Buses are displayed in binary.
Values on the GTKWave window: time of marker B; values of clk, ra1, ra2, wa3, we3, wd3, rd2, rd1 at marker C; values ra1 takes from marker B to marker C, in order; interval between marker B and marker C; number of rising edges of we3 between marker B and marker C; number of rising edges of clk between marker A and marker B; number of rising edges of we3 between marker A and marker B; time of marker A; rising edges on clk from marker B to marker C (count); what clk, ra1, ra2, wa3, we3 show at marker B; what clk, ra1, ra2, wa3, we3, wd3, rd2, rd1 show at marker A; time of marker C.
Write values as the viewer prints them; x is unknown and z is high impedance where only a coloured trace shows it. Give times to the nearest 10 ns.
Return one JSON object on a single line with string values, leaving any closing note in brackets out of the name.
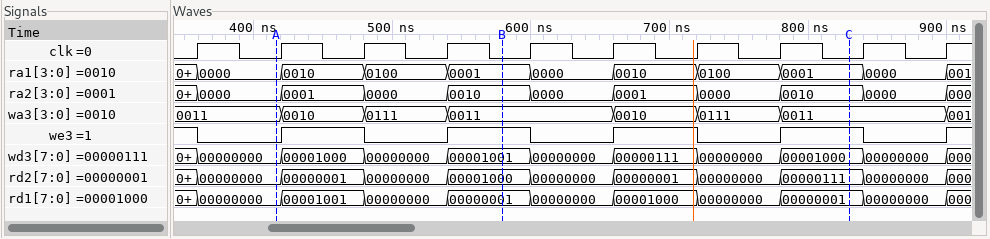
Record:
{"time of marker B": "580 ns", "values of clk, ra1, ra2, wa3, we3, wd3, rd2, rd1 at marker C": "clk=0, ra1=0001, ra2=0010, wa3=0011, we3=1, wd3=00001000, rd2=00000111, rd1=00000001", "values ra1 takes from marker B to marker C, in order": "0001, 0000, 0010, 0100, 0001", "interval between marker B and marker C": "250 ns", "number of rising edges of we3 between marker B and marker C": "2", "number of rising edges of clk between marker A and marker B": "3", "number of rising edges of we3 between marker A and marker B": "2", "time of marker A": "420 ns", "rising edges on clk from marker B to marker C": "4", "what clk, ra1, ra2, wa3, we3 show at marker B": "clk=0, ra1=0001, ra2=0010, wa3=0011, we3=1", "what clk, ra1, ra2, wa3, we3, wd3, rd2, rd1 show at marker A": "clk=0, ra1=0000, ra2=0000, wa3=0011, we3=0, wd3=00000000, rd2=00000000, rd1=00000000", "time of marker C": "830 ns"}
